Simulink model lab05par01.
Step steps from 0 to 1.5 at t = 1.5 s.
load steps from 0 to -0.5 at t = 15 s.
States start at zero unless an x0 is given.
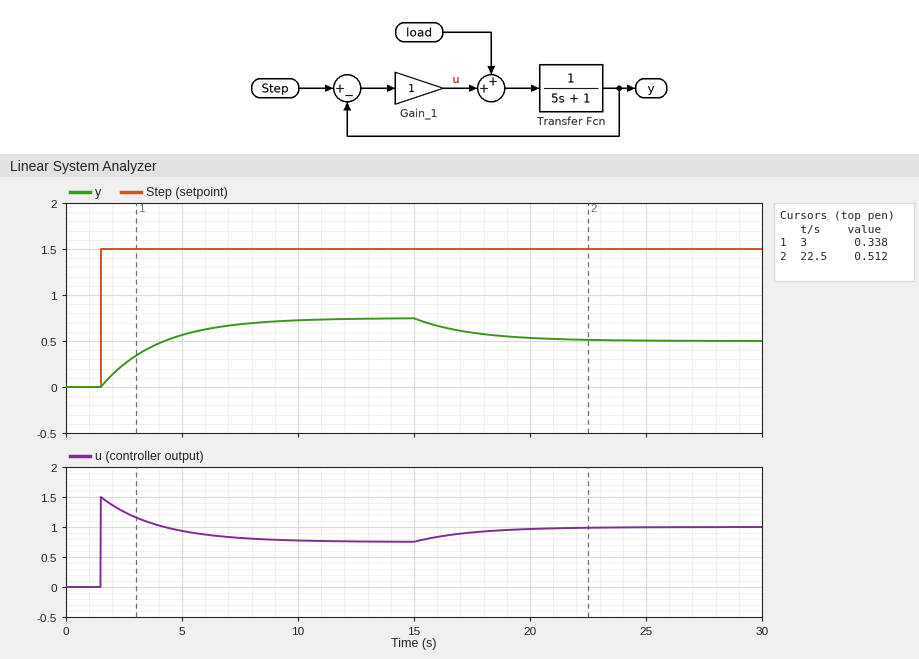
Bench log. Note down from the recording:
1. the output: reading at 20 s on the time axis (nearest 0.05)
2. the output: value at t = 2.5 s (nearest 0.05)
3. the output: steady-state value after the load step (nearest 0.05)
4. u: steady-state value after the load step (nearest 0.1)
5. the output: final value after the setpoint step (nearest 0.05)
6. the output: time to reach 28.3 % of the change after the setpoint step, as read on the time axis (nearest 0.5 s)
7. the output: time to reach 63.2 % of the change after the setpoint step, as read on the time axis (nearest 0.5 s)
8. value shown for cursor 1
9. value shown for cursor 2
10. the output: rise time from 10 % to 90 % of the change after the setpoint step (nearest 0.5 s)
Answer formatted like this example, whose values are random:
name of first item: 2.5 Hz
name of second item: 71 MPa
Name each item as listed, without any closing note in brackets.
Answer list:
the output: reading at 20 s on the time axis: 0.55
the output: value at t = 2.5 s: 0.25
the output: steady-state value after the load step: 0.50
u: steady-state value after the load step: 1.0
the output: final value after the setpoint step: 0.75
the output: time to reach 28.3 % of the change after the setpoint step, as read on the time axis: 2.5 s
the output: time to reach 63.2 % of the change after the setpoint step, as read on the time axis: 4.0 s
value shown for cursor 1: 0.338
value shown for cursor 2: 0.512
the output: rise time from 10 % to 90 % of the change after the setpoint step: 5.5 s
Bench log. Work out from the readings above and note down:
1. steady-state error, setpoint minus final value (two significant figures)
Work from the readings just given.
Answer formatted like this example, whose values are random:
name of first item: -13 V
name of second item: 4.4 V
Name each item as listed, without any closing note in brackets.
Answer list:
steady-state error, setpoint minus final value: 0.75
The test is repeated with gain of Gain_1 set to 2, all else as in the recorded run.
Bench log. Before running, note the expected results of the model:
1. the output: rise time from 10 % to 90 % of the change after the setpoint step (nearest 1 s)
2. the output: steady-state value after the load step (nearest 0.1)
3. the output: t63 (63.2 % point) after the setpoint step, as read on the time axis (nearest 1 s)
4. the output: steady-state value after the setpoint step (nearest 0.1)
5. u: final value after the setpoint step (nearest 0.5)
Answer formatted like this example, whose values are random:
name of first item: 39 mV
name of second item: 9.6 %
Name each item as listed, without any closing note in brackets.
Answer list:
the output: rise time from 10 % to 90 % of the change after the setpoint step: 4 s
the output: steady-state value after the load step: 0.8
the output: t63 (63.2 % point) after the setpoint step, as read on the time axis: 3 s
the output: steady-state value after the setpoint step: 1.0
u: final value after the setpoint step: 1.0
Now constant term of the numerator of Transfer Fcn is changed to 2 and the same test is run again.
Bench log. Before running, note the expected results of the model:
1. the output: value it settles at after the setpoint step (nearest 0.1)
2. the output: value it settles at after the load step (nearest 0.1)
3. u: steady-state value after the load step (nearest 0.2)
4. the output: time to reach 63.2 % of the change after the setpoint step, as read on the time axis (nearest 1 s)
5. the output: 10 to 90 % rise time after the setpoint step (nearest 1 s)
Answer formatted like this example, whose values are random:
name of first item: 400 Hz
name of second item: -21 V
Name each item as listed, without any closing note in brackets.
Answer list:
the output: value it settles at after the setpoint step: 1.0
the output: value it settles at after the load step: 0.7
u: steady-state value after the load step: 0.8
the output: time to reach 63.2 % of the change after the setpoint step, as read on the time axis: 3 s
the output: 10 to 90 % rise time after the setpoint step: 4 s
